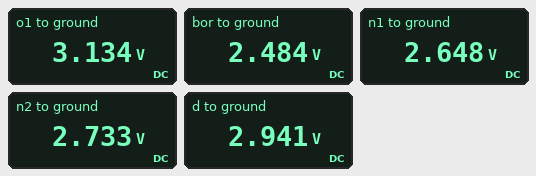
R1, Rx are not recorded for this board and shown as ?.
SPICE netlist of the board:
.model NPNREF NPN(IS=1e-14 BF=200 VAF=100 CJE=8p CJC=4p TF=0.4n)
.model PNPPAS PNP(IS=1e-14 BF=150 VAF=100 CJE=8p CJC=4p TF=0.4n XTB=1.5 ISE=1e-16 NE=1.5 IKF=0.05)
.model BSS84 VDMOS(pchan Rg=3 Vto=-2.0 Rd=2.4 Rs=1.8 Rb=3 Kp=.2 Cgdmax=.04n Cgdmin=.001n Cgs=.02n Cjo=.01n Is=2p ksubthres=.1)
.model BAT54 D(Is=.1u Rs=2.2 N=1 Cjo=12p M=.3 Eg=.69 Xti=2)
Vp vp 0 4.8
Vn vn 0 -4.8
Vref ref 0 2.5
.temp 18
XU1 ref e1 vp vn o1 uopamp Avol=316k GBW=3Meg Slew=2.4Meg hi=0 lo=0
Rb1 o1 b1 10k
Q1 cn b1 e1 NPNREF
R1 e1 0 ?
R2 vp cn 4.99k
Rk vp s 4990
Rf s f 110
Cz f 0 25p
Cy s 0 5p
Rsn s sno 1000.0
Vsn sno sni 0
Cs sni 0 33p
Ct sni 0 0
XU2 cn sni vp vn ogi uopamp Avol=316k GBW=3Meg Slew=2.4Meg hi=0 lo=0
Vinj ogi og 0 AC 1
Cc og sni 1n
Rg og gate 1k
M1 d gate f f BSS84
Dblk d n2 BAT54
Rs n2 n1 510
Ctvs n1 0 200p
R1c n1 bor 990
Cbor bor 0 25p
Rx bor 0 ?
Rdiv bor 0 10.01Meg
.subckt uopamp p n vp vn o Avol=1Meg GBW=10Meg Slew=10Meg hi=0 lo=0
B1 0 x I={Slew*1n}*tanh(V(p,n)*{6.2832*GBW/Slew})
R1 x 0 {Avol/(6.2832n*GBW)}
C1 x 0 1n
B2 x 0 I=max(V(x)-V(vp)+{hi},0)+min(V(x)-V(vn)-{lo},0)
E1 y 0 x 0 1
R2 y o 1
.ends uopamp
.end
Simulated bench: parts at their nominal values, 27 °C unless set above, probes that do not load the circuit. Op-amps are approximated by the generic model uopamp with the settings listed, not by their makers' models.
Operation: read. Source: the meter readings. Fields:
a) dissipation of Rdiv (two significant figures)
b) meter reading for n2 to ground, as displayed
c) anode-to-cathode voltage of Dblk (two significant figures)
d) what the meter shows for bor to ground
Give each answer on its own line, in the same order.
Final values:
620 nW
2.733 V
210 mV
2.484 V
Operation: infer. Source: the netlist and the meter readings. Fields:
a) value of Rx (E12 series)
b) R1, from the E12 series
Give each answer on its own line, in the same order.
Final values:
15 kΩ
15 kΩ
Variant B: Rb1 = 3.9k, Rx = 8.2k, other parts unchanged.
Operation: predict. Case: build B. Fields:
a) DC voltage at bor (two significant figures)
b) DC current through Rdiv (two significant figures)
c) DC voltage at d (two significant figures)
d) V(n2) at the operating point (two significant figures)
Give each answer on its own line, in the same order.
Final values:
1.4 V
140 nA
1.8 V
1.6 V
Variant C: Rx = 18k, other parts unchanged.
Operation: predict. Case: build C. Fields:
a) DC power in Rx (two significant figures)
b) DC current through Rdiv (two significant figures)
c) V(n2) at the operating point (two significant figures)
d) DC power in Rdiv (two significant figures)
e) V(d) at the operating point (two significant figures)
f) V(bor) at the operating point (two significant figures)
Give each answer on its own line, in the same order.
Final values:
490 µW
300 nA
3.2 V
890 nW
3.4 V
3.0 V
